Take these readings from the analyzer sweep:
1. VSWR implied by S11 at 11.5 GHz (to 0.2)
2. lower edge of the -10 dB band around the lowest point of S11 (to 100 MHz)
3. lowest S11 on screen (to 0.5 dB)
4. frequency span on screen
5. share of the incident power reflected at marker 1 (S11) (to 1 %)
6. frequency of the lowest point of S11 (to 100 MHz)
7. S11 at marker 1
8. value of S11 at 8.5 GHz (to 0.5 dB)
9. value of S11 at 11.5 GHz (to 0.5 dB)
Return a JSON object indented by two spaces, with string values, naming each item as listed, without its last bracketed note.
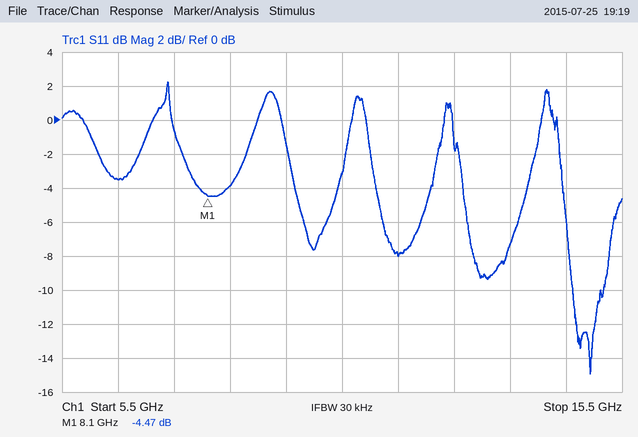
{
  "VSWR implied by S11 at 11.5 GHz": "2.4",
  "lower edge of the -10 dB band around the lowest point of S11": "14.6 GHz",
  "lowest S11 on screen": "-15.0 dB",
  "frequency span on screen": "10 GHz",
  "share of the incident power reflected at marker 1 (S11)": "36 %",
  "frequency of the lowest point of S11": "14.9 GHz",
  "S11 at marker 1": "-4.47 dB",
  "value of S11 at 8.5 GHz": "-4.0 dB",
  "value of S11 at 11.5 GHz": "-8.0 dB"
}
